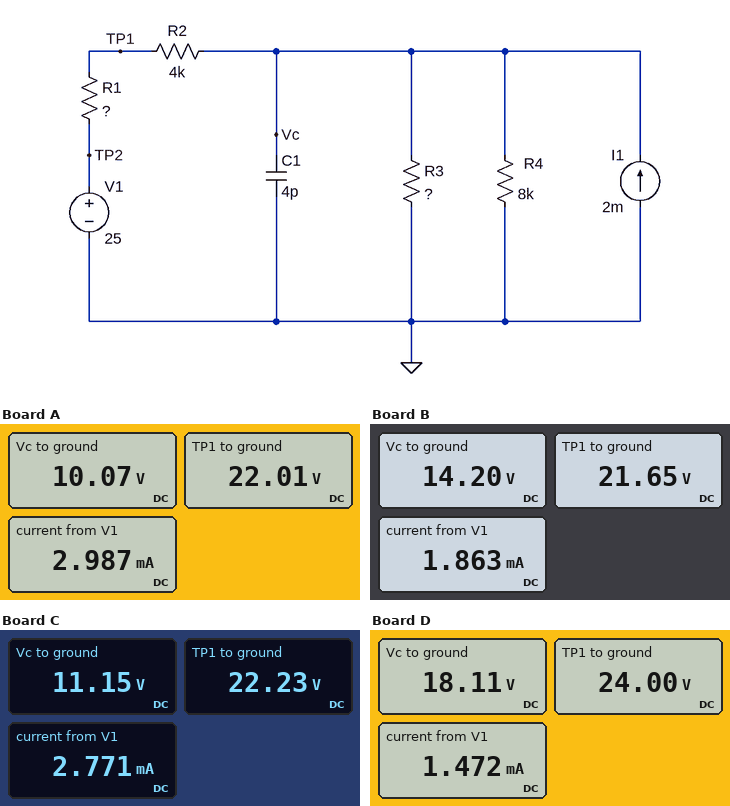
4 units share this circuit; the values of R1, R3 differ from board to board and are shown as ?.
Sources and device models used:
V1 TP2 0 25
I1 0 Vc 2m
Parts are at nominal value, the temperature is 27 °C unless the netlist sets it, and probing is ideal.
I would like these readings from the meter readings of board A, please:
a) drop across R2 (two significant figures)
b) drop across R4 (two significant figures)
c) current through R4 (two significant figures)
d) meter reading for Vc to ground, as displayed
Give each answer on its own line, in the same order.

12 V
10 V
1.3 mA
10.07 V
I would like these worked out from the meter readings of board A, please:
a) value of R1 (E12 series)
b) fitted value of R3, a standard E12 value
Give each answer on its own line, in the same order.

1 kΩ
2.7 kΩ
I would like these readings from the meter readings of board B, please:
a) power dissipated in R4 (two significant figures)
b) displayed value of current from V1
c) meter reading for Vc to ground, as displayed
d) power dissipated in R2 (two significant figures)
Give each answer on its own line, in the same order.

25 mW
1.863 mA
14.20 V
14 mW
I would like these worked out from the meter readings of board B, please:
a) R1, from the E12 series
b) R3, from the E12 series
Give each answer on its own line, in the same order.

1.8 kΩ
6.8 kΩ
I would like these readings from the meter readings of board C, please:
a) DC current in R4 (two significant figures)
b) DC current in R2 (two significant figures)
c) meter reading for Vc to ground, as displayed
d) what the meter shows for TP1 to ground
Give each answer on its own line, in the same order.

1.4 mA
2.8 mA
11.15 V
22.23 V
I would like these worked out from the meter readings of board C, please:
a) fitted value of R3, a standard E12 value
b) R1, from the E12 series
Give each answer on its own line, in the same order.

3.3 kΩ
1 kΩ
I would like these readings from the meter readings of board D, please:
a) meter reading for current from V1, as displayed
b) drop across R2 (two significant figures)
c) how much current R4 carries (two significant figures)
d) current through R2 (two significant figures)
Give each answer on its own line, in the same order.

1.472 mA
5.9 V
2.3 mA
1.5 mA
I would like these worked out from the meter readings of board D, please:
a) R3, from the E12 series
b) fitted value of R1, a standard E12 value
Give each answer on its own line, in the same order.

15 kΩ
680 Ω
